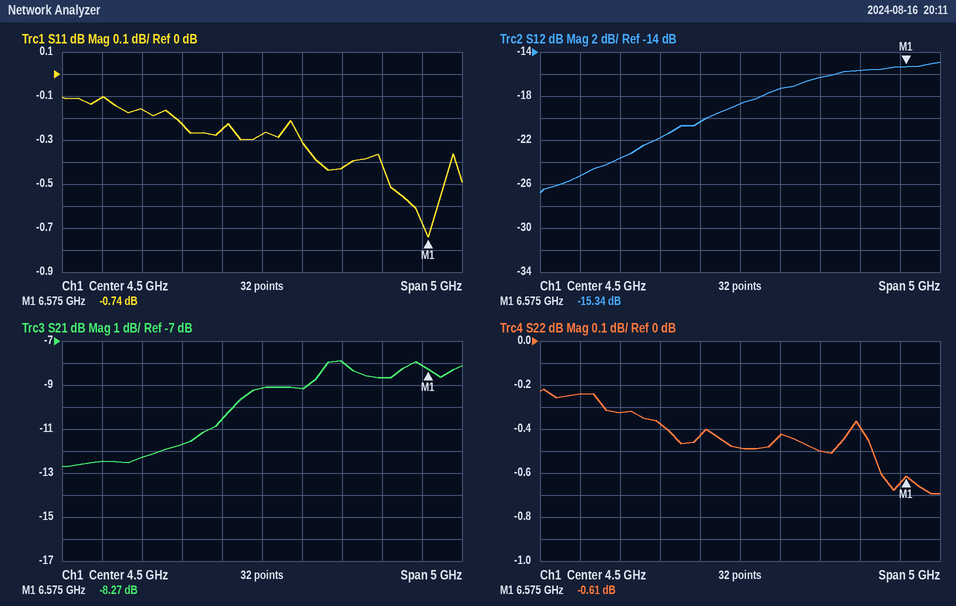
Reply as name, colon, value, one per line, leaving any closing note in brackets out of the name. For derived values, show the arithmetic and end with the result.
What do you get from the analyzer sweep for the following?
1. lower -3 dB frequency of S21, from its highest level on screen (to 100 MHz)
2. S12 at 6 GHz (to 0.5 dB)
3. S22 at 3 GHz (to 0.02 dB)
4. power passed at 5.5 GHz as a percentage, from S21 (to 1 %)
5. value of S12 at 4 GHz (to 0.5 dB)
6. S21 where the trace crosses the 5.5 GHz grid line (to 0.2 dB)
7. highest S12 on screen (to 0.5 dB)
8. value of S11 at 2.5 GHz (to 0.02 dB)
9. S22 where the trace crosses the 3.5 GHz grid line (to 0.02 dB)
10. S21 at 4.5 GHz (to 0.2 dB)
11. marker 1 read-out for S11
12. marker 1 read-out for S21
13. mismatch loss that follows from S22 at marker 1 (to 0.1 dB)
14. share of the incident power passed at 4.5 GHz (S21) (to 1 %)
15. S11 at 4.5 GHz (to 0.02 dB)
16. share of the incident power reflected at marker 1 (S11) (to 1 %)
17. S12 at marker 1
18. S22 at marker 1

lower -3 dB frequency of S21, from its highest level on screen: 3.9 GHz
S12 at 6 GHz: -15.5 dB
S22 at 3 GHz: -0.32 dB
power passed at 5.5 GHz as a percentage, from S21: 10^(-8/10) ≈ 16 %
value of S12 at 4 GHz: -20.5 dB
S21 where the trace crosses the 5.5 GHz grid line: -8.0 dB
highest S12 on screen: -15.0 dB
value of S11 at 2.5 GHz: -0.10 dB
S22 where the trace crosses the 3.5 GHz grid line: -0.38 dB
S21 at 4.5 GHz: -9.2 dB
marker 1 read-out for S11: -0.74 dB
marker 1 read-out for S21: -8.27 dB
mismatch loss that follows from S22 at marker 1: −10 log10(1 − 10^(-0.61/10)) ≈ 8.8 dB
share of the incident power passed at 4.5 GHz (S21): 10^(-9.2/10) ≈ 12 %
S11 at 4.5 GHz: -0.28 dB
share of the incident power reflected at marker 1 (S11): 10^(-0.74/10) ≈ 84 %
S12 at marker 1: -15.34 dB
S22 at marker 1: -0.61 dB
